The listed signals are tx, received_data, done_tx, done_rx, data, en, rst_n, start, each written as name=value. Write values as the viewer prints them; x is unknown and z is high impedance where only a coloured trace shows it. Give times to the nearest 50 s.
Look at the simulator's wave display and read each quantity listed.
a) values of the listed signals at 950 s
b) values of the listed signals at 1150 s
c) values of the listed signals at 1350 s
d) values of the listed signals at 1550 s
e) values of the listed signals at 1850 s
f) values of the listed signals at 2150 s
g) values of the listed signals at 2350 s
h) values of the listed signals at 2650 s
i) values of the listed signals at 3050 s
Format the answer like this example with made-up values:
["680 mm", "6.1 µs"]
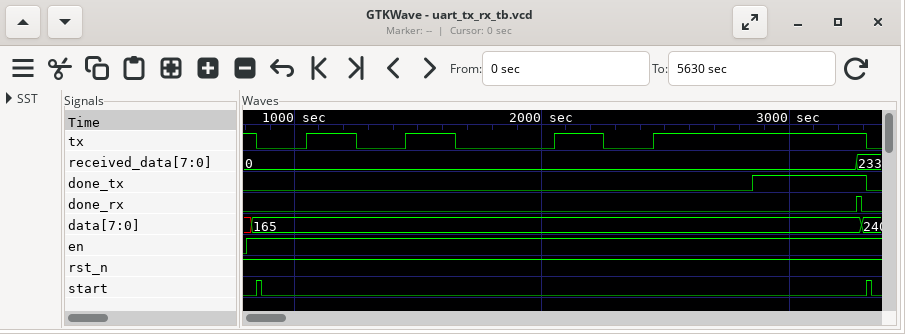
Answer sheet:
["tx=0, received_data=0, done_tx=0, done_rx=0, data=165, en=1, rst_n=1, start=0", "tx=1, received_data=0, done_tx=0, done_rx=0, data=165, en=1, rst_n=1, start=0", "tx=0, received_data=0, done_tx=0, done_rx=0, data=165, en=1, rst_n=1, start=0", "tx=1, received_data=0, done_tx=0, done_rx=0, data=165, en=1, rst_n=1, start=0", "tx=0, received_data=0, done_tx=0, done_rx=0, data=165, en=1, rst_n=1, start=0", "tx=1, received_data=0, done_tx=0, done_rx=0, data=165, en=1, rst_n=1, start=0", "tx=0, received_data=0, done_tx=0, done_rx=0, data=165, en=1, rst_n=1, start=0", "tx=1, received_data=0, done_tx=0, done_rx=0, data=165, en=1, rst_n=1, start=0", "tx=1, received_data=0, done_tx=1, done_rx=0, data=165, en=1, rst_n=1, start=0"]
